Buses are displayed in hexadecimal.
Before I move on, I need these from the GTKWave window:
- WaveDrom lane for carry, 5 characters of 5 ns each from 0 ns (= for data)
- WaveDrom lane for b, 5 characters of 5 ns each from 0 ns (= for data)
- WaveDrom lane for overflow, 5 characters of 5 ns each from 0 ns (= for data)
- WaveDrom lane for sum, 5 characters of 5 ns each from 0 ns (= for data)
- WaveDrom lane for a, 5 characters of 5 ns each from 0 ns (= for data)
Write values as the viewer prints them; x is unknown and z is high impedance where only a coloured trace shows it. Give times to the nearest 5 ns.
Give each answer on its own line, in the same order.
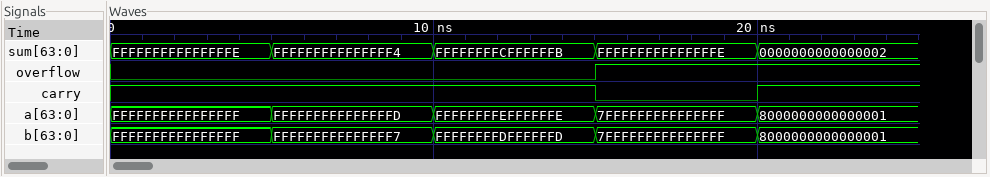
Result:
{name: 'carry', wave: '1..01'}
{name: 'b', wave: '=====', data: 'FFFFFFFFFFFFFFFF FFFFFFFFFFFFFFF7 FFFFFFFFDFFFFFFD 7FFFFFFFFFFFFFFF 8000000000000001'}
{name: 'overflow', wave: '0..1.'}
{name: 'sum', wave: '=====', data: 'FFFFFFFFFFFFFFFE FFFFFFFFFFFFFFF4 FFFFFFFFCFFFFFFB FFFFFFFFFFFFFFFE 0000000000000002'}
{name: 'a', wave: '=====', data: 'FFFFFFFFFFFFFFFF FFFFFFFFFFFFFFFD FFFFFFFFEFFFFFFE 7FFFFFFFFFFFFFFF 8000000000000001'}
